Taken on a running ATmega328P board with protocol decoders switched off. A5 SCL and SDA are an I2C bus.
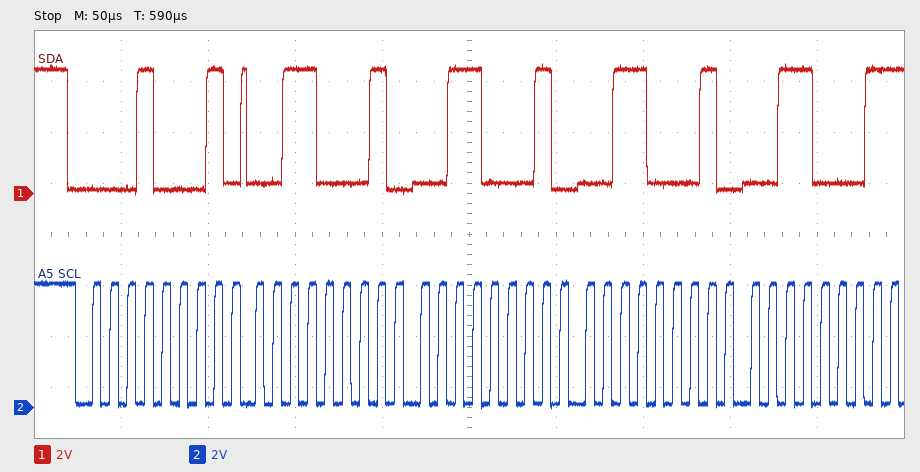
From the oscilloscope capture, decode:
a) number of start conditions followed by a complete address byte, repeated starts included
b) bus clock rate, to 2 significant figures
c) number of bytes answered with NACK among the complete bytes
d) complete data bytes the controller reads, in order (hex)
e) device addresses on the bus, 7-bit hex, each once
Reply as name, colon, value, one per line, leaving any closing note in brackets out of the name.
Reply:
number of start conditions followed by a complete address byte, repeated starts included: 1
bus clock rate, to 2 significant figures: 100 kHz
number of bytes answered with NACK among the complete bytes: 1
complete data bytes the controller reads, in order: 31 31 31 31
device addresses on the bus, 7-bit hex, each once: 0x08
